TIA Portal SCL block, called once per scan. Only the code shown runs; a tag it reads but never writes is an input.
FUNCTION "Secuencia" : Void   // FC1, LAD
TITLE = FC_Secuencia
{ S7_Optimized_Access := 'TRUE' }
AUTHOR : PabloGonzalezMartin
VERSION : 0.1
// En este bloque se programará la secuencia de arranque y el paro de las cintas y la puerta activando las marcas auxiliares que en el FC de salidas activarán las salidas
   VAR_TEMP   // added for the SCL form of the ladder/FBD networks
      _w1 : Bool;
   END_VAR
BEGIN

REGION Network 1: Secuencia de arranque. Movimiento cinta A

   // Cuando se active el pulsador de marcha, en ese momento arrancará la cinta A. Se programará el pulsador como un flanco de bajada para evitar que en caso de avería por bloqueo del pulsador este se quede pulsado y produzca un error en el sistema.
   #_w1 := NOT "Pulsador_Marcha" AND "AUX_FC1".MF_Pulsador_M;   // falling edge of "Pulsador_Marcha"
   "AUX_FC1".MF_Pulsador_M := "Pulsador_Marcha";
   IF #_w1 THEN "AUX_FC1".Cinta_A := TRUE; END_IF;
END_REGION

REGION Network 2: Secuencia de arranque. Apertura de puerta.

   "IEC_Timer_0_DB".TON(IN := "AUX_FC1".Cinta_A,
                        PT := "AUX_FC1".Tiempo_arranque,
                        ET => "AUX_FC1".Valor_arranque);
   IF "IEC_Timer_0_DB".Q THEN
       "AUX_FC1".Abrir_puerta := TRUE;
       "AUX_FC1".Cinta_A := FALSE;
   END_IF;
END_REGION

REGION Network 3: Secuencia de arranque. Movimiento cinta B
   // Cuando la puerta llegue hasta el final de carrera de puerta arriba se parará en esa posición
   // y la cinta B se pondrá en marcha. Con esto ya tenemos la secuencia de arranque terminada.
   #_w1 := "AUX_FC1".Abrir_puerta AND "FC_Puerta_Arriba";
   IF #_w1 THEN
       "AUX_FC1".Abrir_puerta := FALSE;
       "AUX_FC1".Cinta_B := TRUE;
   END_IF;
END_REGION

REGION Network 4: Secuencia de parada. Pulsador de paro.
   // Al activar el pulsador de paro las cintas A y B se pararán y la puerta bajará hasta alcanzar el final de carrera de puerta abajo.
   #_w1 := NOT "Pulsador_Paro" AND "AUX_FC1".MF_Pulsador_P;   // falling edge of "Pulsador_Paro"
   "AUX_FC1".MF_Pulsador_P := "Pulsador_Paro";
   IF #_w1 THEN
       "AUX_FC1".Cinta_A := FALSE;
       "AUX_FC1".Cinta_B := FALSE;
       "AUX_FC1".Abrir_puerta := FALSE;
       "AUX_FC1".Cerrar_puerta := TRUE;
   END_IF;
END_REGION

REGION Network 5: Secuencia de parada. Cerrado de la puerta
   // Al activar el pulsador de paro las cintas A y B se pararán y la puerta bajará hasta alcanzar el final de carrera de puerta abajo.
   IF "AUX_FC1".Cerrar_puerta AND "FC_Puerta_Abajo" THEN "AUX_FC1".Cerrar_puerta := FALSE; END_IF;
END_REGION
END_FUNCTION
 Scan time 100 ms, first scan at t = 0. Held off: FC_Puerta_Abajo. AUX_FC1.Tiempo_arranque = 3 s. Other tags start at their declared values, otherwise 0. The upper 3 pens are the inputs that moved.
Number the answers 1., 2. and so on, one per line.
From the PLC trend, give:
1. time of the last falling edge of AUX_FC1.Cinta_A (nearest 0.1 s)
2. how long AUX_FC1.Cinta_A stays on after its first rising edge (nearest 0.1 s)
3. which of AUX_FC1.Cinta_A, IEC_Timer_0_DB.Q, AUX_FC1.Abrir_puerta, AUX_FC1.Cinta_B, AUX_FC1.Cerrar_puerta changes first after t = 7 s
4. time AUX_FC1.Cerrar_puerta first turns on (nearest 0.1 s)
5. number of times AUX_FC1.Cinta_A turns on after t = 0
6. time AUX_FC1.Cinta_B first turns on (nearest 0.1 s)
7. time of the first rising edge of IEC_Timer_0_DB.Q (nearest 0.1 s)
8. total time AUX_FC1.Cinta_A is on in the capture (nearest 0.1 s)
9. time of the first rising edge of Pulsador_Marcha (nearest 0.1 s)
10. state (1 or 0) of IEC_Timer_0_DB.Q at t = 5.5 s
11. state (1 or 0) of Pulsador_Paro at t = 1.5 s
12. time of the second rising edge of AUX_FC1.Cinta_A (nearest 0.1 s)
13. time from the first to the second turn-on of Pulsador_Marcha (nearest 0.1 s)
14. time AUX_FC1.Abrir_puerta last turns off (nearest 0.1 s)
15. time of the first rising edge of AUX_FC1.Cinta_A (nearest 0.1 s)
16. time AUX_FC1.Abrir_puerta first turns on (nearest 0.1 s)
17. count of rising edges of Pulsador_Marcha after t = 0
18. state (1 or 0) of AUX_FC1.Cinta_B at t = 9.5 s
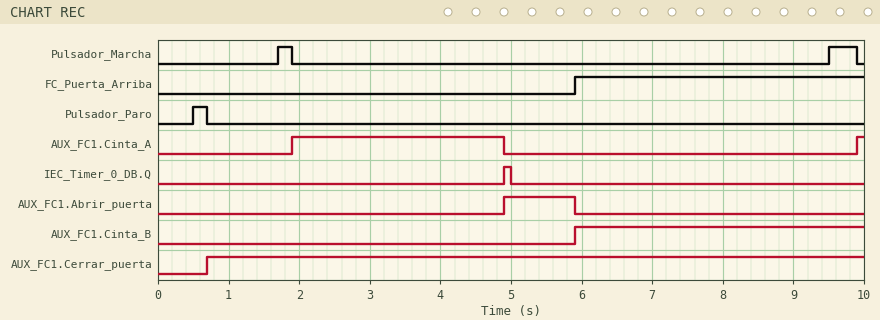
1. 4.9 s
2. 3.0 s
3. AUX_FC1.Cinta_A
4. 0.7 s
5. 2
6. 5.9 s
7. 4.9 s
8. 3.1 s
9. 1.7 s
10. 0
11. 0
12. 9.9 s
13. 7.8 s
14. 5.9 s
15. 1.9 s
16. 4.9 s
17. 2
18. 1
